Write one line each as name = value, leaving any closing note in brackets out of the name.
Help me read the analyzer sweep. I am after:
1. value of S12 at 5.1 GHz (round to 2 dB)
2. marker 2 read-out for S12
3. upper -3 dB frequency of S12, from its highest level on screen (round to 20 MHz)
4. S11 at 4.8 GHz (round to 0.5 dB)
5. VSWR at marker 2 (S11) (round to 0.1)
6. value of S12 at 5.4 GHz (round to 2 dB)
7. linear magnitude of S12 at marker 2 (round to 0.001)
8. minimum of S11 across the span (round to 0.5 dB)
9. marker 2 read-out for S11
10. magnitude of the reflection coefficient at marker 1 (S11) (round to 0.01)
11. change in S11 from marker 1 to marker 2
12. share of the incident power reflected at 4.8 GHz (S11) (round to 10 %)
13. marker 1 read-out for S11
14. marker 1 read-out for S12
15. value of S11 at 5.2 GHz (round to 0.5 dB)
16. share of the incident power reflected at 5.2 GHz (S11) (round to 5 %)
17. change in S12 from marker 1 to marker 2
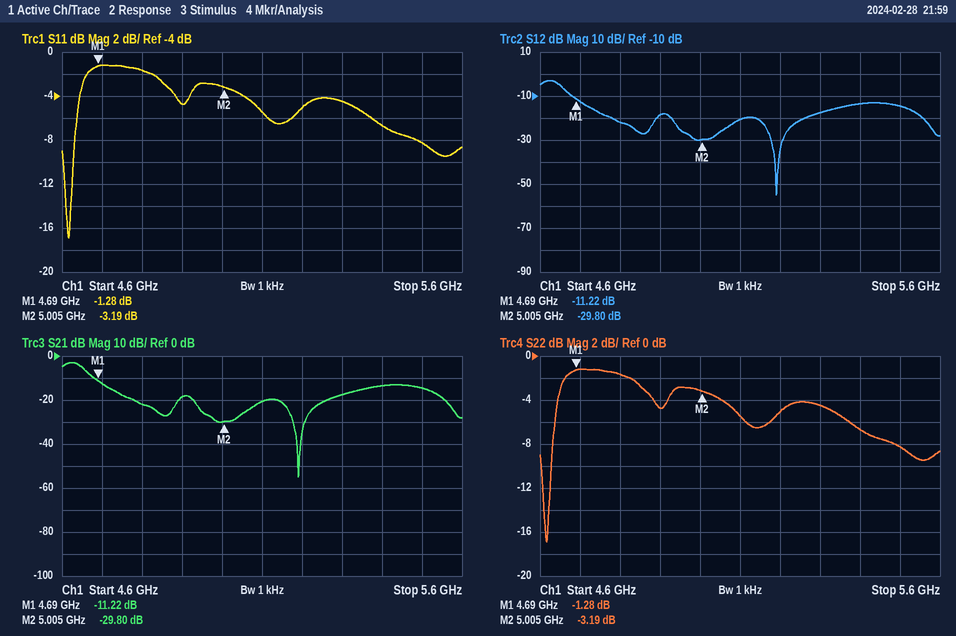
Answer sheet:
value of S12 at 5.1 GHz = -20 dB
marker 2 read-out for S12 = -29.80 dB
upper -3 dB frequency of S12, from its highest level on screen = 4.66 GHz
S11 at 4.8 GHz = -1.5 dB
VSWR at marker 2 (S11) = 5.5
value of S12 at 5.4 GHz = -14 dB
linear magnitude of S12 at marker 2 = 0.032
minimum of S11 across the span = -17.0 dB
marker 2 read-out for S11 = -3.19 dB
magnitude of the reflection coefficient at marker 1 (S11) = 0.86
change in S11 from marker 1 to marker 2 = -1.91 dB
share of the incident power reflected at 4.8 GHz (S11) = 70 %
marker 1 read-out for S11 = -1.28 dB
marker 1 read-out for S12 = -11.22 dB
value of S11 at 5.2 GHz = -5.0 dB
share of the incident power reflected at 5.2 GHz (S11) = 30 %
change in S12 from marker 1 to marker 2 = -18.58 dB
